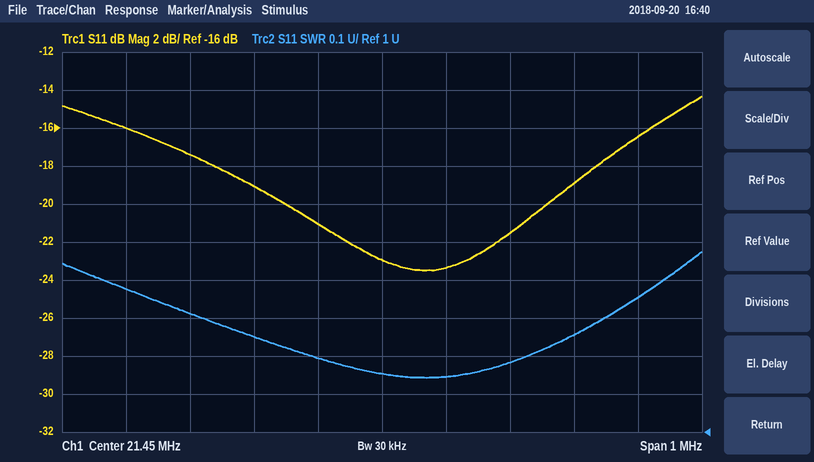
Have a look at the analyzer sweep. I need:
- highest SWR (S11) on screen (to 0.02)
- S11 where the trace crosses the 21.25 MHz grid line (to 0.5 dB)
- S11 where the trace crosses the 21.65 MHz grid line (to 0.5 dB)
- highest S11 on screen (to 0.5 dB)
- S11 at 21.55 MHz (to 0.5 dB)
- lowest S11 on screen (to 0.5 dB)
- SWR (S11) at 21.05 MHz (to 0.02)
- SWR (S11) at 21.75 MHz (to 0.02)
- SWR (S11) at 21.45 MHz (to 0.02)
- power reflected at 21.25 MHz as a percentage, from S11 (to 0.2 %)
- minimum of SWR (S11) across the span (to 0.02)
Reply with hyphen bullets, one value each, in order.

- 1.48
- -19.0 dB
- -21.5 dB
- -14.5 dB
- -23.5 dB
- -23.5 dB
- 1.38
- 1.26
- 1.16
- 1.2 %
- 1.14
